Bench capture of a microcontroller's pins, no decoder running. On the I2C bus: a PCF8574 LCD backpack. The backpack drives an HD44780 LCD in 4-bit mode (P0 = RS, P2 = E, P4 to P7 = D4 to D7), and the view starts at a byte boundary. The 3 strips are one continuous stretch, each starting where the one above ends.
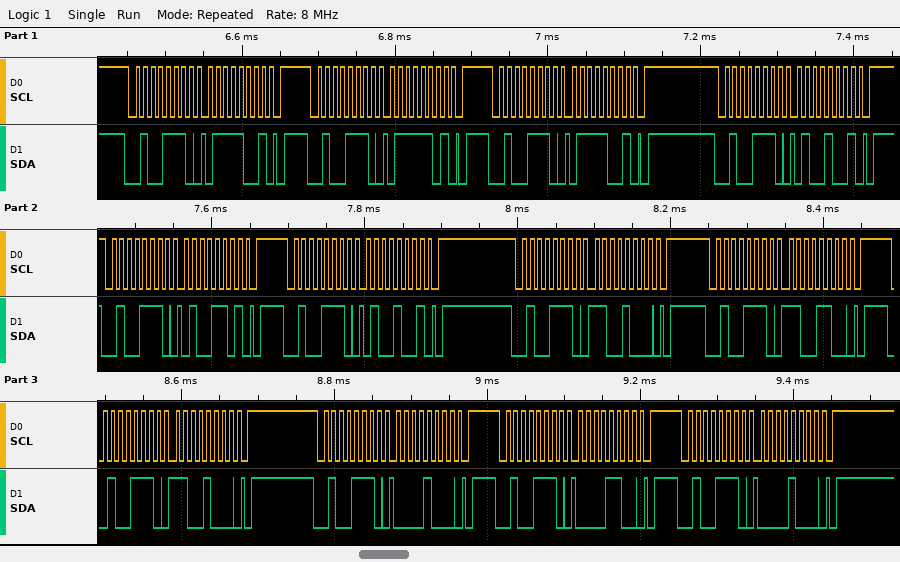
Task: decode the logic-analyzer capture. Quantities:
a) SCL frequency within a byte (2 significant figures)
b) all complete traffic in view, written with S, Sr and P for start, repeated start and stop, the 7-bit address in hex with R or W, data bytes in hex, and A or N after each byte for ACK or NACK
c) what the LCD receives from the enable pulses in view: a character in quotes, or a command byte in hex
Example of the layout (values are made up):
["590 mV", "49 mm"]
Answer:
["100 kHz", "S 27W A 79 A P S 27W A 7D A P S 27W A 79 A P S 27W A 49 A P S 27W A 4D A P S 27W A 49 A P S 27W A C8 A P S 27W A CC A P S 27W A C8 A P S 27W A 08 A P S 27W A 0C A P S 27W A 08 A P", "'t' 0xC0"]
